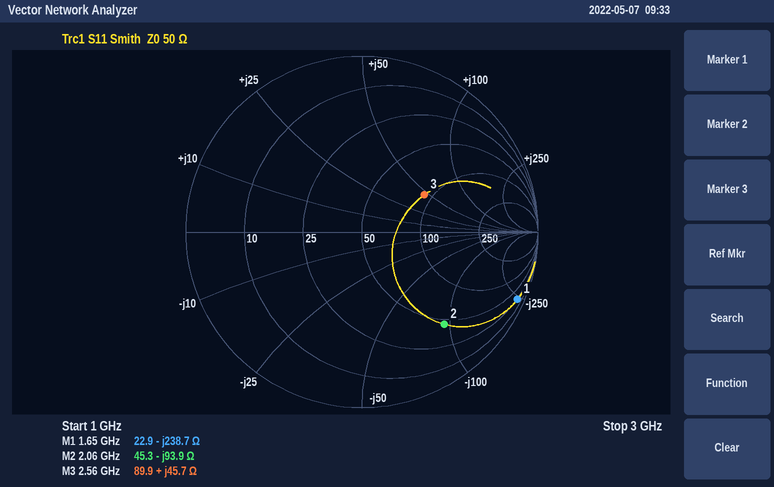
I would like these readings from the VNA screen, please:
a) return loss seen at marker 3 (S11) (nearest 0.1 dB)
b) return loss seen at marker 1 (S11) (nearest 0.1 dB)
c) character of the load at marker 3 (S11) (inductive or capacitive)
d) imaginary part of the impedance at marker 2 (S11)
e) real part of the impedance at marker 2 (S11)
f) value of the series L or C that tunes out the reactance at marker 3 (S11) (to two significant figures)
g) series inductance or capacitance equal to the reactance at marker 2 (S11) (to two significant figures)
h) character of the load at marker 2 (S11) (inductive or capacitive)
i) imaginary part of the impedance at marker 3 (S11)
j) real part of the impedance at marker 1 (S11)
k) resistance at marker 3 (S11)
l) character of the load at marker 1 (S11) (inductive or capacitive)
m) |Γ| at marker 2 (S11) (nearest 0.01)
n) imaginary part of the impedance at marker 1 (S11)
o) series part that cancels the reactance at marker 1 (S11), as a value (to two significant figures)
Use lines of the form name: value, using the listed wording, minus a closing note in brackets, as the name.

return loss seen at marker 3 (S11): 7.7 dB
return loss seen at marker 1 (S11): 0.3 dB
character of the load at marker 3 (S11): inductive
imaginary part of the impedance at marker 2: -93.9 Ω
real part of the impedance at marker 2: 45.3 Ω
value of the series L or C that tunes out the reactance at marker 3 (S11): 1.4 pF
series inductance or capacitance equal to the reactance at marker 2 (S11): 820 fF
character of the load at marker 2 (S11): capacitive
imaginary part of the impedance at marker 3: +45.7 Ω
real part of the impedance at marker 1: 22.9 Ω
resistance at marker 3: 89.9 Ω
character of the load at marker 1 (S11): capacitive
|Γ| at marker 2 (S11): 0.70
imaginary part of the impedance at marker 1: -238.7 Ω
series part that cancels the reactance at marker 1 (S11), as a value: 23 nH
